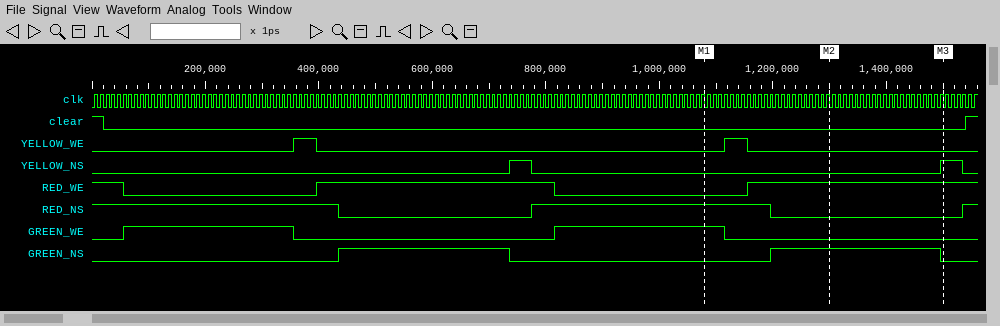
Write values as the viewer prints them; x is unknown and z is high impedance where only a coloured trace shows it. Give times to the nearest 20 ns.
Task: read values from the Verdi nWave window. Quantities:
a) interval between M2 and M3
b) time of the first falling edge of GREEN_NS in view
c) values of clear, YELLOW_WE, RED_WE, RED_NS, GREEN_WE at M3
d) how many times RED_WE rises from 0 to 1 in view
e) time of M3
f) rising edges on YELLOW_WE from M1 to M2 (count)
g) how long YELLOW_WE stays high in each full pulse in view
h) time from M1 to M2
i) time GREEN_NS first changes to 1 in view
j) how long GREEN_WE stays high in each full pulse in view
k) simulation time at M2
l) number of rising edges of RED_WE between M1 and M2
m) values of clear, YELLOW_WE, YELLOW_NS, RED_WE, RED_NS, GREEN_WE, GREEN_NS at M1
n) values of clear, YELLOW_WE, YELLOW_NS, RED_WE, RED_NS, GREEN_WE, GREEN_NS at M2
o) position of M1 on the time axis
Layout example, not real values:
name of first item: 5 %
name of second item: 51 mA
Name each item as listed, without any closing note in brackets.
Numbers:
interval between M2 and M3: 200 ns
time of the first falling edge of GREEN_NS in view: 740 ns
values of clear, YELLOW_WE, RED_WE, RED_NS, GREEN_WE at M3: clear=0, YELLOW_WE=0, RED_WE=1, RED_NS=0, GREEN_WE=0
how many times RED_WE rises from 0 to 1 in view: 2
time of M3: 1500 ns
rising edges on YELLOW_WE from M1 to M2: 1
how long YELLOW_WE stays high in each full pulse in view: 40 ns, 40 ns
time from M1 to M2: 220 ns
time GREEN_NS first changes to 1 in view: 440 ns
how long GREEN_WE stays high in each full pulse in view: 300 ns, 300 ns
simulation time at M2: 1300 ns
number of rising edges of RED_WE between M1 and M2: 1
values of clear, YELLOW_WE, YELLOW_NS, RED_WE, RED_NS, GREEN_WE, GREEN_NS at M1: clear=0, YELLOW_WE=0, YELLOW_NS=0, RED_WE=0, RED_NS=1, GREEN_WE=1, GREEN_NS=0
values of clear, YELLOW_WE, YELLOW_NS, RED_WE, RED_NS, GREEN_WE, GREEN_NS at M2: clear=0, YELLOW_WE=0, YELLOW_NS=0, RED_WE=1, RED_NS=0, GREEN_WE=0, GREEN_NS=1
position of M1 on the time axis: 1080 ns
